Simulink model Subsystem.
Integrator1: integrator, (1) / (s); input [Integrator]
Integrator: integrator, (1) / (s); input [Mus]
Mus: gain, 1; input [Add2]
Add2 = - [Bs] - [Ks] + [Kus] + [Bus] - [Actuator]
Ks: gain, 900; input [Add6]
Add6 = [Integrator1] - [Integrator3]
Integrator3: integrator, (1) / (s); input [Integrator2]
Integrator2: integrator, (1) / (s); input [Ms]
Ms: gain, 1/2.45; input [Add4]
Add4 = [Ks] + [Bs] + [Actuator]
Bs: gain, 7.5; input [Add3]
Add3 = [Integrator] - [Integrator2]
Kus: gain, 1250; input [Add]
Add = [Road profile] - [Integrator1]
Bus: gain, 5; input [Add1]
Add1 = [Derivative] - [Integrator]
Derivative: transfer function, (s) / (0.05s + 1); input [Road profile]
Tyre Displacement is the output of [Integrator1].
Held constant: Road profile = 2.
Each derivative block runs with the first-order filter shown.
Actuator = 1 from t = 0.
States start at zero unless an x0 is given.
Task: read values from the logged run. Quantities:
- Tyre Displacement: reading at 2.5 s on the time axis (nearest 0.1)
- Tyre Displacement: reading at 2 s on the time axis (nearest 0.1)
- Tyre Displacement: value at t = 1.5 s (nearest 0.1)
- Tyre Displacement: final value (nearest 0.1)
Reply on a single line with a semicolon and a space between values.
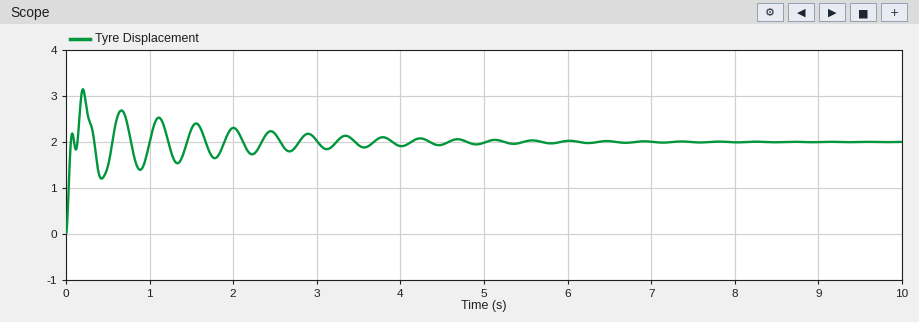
2.2; 2.3; 2.3; 2.0
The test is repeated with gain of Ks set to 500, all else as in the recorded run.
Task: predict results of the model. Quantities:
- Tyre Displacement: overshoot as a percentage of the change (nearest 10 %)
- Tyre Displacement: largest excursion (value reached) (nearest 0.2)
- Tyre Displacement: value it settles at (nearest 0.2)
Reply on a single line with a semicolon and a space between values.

40 %; 2.8; 2.0
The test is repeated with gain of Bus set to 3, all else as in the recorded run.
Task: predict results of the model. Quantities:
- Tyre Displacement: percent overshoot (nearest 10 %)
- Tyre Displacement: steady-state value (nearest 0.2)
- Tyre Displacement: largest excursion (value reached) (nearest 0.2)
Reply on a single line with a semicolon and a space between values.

60 %; 2.0; 3.2
